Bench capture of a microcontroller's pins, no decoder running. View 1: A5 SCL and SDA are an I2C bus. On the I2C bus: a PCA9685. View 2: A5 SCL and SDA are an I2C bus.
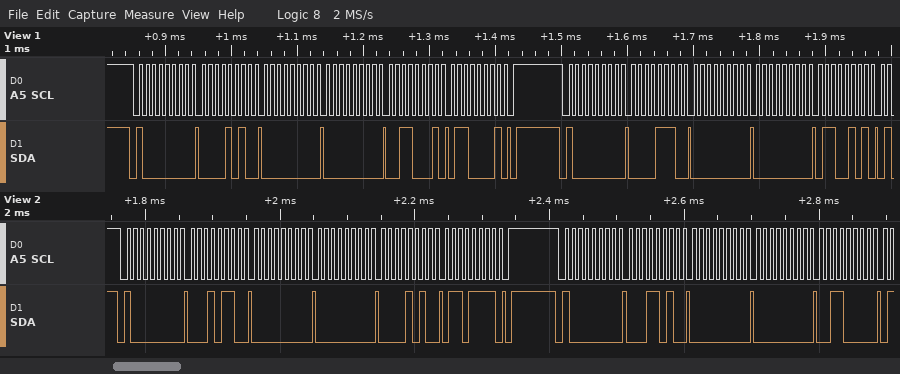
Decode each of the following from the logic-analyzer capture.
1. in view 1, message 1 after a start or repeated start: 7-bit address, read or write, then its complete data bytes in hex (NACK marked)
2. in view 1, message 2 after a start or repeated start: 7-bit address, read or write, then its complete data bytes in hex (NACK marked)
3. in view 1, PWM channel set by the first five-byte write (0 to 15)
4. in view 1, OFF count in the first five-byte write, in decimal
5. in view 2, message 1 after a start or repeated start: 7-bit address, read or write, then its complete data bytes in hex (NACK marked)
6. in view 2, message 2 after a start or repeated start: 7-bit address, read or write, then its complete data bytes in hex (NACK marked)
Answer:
0x40 write: 0A 00 00 31 61
0x40 write: 0E 00 00 65
1
24881
0x40 write: 16 00 00 0A 6F
0x40 write: 1A 00 00 30
